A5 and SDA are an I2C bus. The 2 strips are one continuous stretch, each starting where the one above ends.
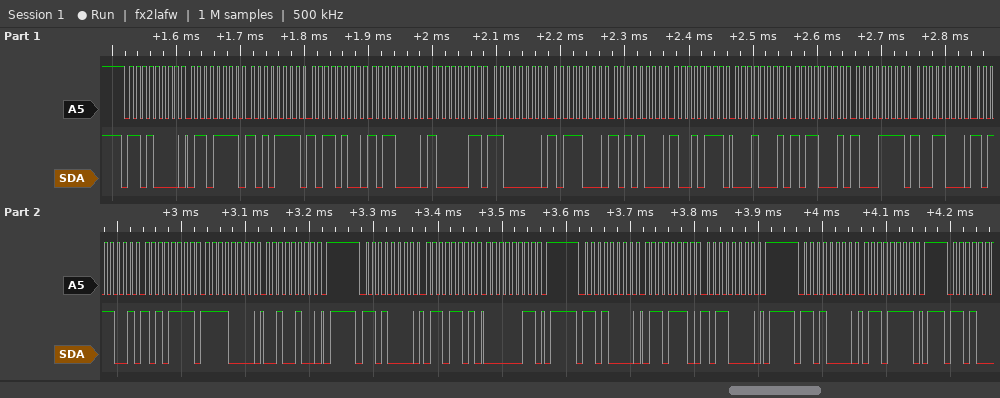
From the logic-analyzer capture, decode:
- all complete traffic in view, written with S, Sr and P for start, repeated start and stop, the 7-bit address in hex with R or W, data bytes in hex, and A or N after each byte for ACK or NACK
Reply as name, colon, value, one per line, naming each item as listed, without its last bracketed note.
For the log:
all complete traffic in view, written with S, Sr and P for start, repeated start and stop, the 7-bit address in hex with R or W, data bytes in hex, and A or N after each byte for ACK or NACK: S 68W A 6F A AF A B4 A B0 A 83 A C0 A B8 A A8 A 97 A 11 A B1 A 8F A 98 A B9 A AF A F0 A 24 A P S 68W A 6D A 03 A P S 68W A 6E A B0 A P S 68W A 6F A P
